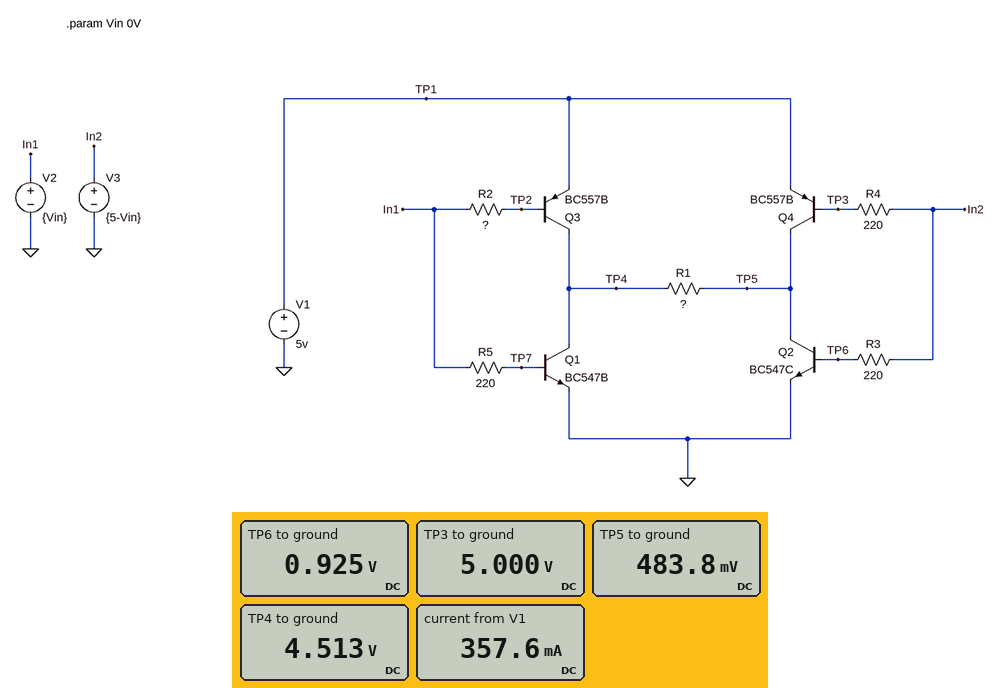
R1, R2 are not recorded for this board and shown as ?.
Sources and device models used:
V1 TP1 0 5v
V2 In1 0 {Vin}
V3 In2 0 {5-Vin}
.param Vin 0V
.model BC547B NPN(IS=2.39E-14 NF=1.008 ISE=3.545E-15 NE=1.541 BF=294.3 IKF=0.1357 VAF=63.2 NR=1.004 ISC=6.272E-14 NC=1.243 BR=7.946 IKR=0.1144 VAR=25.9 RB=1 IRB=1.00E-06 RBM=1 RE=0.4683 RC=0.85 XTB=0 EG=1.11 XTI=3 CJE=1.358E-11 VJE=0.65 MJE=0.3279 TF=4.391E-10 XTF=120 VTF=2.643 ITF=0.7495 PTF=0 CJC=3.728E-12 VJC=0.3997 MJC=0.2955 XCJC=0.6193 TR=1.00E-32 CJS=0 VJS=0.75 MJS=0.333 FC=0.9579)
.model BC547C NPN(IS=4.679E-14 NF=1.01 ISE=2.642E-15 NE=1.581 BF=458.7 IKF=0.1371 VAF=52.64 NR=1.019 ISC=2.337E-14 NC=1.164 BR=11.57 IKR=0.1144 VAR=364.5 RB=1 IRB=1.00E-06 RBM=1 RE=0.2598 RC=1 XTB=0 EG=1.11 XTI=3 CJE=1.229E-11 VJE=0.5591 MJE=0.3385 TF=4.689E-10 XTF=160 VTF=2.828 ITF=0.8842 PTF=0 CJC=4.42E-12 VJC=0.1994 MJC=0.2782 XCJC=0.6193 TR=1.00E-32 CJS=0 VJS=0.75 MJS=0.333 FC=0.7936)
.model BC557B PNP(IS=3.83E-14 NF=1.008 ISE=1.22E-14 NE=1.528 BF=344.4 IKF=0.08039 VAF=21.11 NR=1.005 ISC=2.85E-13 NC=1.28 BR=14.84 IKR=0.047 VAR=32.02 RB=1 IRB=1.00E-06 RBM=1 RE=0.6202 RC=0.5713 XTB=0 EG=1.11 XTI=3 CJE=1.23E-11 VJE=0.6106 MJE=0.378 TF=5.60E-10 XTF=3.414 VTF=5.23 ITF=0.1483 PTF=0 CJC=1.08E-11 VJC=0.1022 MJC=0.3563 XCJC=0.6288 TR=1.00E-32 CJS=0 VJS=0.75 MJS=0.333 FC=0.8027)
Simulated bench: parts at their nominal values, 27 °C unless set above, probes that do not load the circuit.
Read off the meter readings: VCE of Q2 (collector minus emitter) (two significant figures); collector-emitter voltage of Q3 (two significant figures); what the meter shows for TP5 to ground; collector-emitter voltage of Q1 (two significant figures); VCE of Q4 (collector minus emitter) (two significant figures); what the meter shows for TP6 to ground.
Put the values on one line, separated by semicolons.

480 mV; -490 mV; 483.8 mV; 4.5 V; -4.5 V; 0.925 V
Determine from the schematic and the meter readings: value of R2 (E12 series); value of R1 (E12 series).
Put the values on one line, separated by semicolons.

180 Ω; 12 Ω
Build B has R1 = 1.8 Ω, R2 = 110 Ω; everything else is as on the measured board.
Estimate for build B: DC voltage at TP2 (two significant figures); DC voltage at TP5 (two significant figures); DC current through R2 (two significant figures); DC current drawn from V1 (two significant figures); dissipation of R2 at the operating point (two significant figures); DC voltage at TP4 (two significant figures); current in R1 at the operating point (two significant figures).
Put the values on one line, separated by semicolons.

3.5 V; 1.3 V; 32 mA; 920 mA; 110 mW; 2.9 V; 890 mA
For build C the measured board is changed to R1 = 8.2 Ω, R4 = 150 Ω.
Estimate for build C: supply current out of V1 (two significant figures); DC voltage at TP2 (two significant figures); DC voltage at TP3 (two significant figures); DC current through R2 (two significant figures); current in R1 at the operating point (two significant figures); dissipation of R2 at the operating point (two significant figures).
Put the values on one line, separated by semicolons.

470 mA; 3.8 V; 5.0 V; 21 mA; 450 mA; 82 mW
